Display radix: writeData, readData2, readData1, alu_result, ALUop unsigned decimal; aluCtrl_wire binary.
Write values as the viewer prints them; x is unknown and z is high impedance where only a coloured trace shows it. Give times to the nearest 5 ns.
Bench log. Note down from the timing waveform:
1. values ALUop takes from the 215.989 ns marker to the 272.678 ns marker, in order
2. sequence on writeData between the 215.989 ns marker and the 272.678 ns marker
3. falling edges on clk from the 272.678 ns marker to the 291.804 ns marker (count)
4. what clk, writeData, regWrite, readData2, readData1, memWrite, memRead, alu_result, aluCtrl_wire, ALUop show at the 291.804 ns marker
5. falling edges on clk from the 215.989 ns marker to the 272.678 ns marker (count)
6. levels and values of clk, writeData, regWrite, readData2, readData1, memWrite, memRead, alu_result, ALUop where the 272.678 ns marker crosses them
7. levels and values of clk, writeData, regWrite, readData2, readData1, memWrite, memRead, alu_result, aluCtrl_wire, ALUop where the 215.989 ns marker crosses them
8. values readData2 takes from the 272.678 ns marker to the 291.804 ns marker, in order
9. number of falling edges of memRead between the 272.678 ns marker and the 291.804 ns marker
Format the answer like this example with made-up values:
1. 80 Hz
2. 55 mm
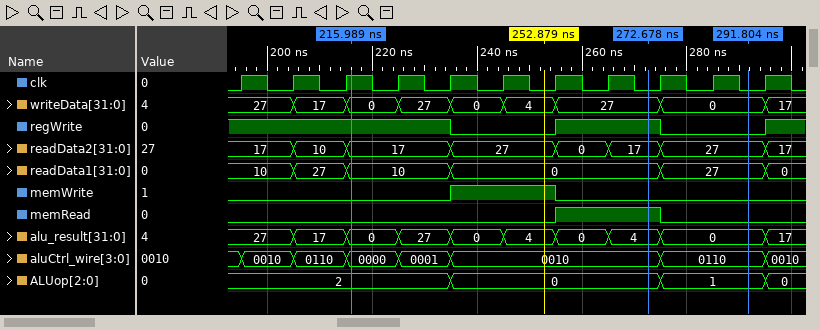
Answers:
1. 2, 0
2. 0, 27, 0, 4, 27
3. 2
4. clk=0, writeData=0, regWrite=0, readData2=27, readData1=27, memWrite=0, memRead=0, alu_result=0, aluCtrl_wire=0110, ALUop=1
5. 6
6. clk=0, writeData=27, regWrite=1, readData2=17, readData1=0, memWrite=0, memRead=1, alu_result=4, ALUop=0
7. clk=1, writeData=0, regWrite=1, readData2=17, readData1=10, memWrite=0, memRead=0, alu_result=0, aluCtrl_wire=0000, ALUop=2
8. 17, 27
9. 1
